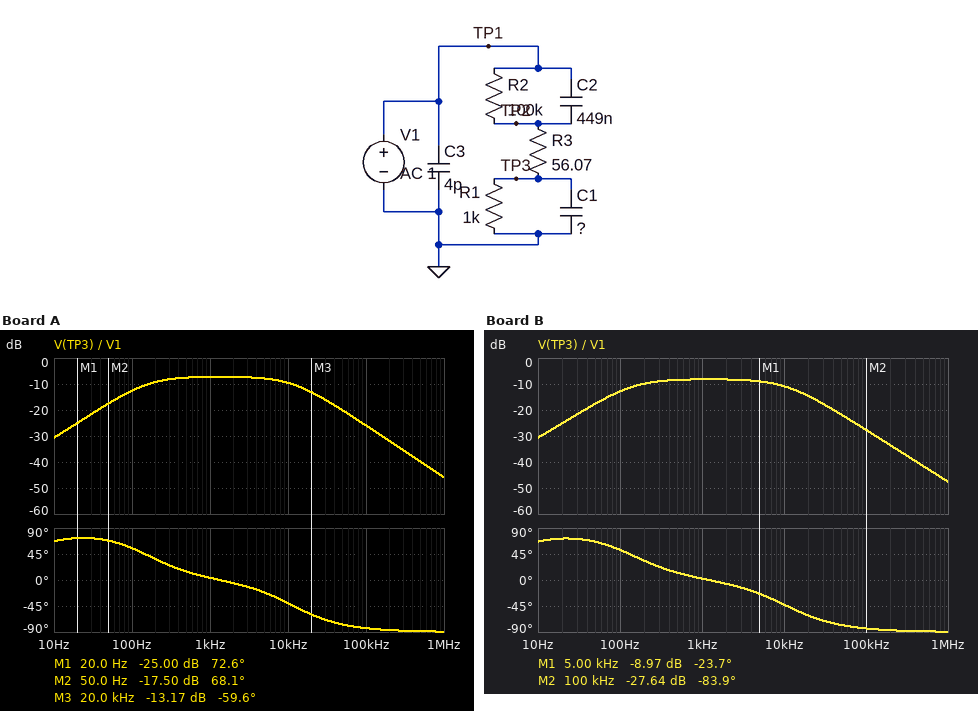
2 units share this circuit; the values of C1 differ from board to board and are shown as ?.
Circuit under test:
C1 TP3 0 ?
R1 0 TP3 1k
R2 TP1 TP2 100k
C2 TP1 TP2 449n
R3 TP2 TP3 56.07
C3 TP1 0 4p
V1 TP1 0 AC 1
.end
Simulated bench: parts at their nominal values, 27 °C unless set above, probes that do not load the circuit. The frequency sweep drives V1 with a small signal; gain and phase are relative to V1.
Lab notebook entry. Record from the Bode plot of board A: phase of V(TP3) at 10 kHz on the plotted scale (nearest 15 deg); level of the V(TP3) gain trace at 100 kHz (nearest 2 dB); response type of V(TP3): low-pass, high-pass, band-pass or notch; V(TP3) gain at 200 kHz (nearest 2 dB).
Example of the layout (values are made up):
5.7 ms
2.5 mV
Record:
-45 deg
-26 dB
band-pass
-32 dB
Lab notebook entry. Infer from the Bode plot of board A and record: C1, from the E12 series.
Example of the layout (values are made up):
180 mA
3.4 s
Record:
560 nF
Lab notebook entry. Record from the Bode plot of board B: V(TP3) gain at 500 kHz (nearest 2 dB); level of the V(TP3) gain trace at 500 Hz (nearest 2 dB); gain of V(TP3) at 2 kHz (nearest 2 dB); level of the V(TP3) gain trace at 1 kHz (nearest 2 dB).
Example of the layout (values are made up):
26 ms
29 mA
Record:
-42 dB
-8 dB
-8 dB
-8 dB
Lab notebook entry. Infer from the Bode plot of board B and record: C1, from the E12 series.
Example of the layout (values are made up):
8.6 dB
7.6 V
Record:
680 nF
